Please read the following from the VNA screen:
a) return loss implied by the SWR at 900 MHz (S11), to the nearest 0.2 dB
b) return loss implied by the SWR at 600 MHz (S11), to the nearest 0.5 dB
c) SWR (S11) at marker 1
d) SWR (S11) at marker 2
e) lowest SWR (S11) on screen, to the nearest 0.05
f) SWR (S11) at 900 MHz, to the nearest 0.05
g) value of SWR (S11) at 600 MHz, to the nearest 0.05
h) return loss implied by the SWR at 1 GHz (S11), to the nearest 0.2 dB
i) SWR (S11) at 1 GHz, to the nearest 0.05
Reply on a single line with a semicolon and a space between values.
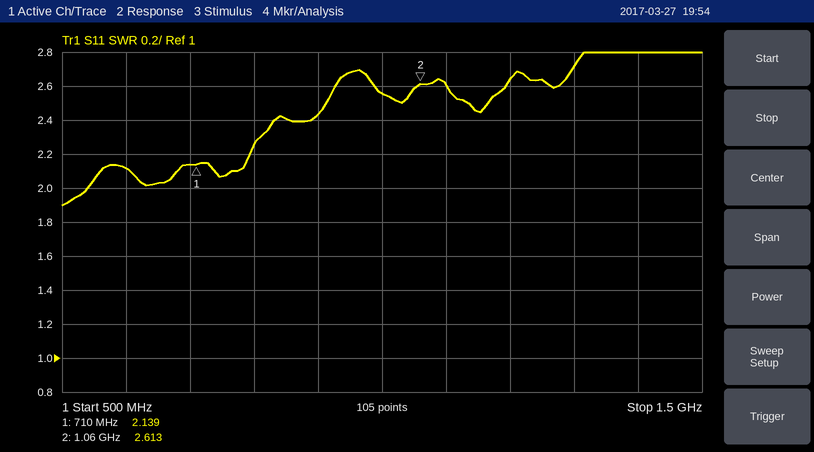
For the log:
7.6 dB; 9.0 dB; 2.139; 2.613; 1.90; 2.45; 2.10; 7.2 dB; 2.55
